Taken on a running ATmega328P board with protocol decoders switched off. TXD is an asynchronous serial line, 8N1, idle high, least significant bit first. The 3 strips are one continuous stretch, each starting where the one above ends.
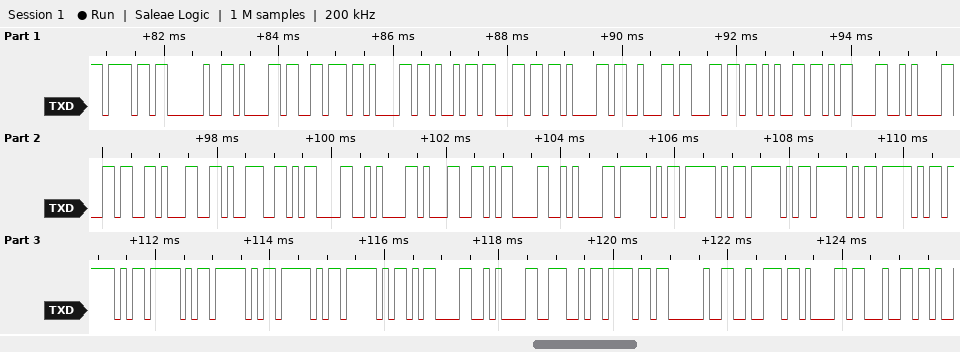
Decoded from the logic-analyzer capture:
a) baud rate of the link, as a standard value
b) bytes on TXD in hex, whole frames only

9600 baud
6F 20 61 76 61 69 6C 61 62 6C 65 0D 0A 36 31 39 0D 0A 31 0D 0A 5F 5F 5F 5F 5F 5F 5F 5F 5F 5F 0D 0A 4E 6F 20 72 61 64
